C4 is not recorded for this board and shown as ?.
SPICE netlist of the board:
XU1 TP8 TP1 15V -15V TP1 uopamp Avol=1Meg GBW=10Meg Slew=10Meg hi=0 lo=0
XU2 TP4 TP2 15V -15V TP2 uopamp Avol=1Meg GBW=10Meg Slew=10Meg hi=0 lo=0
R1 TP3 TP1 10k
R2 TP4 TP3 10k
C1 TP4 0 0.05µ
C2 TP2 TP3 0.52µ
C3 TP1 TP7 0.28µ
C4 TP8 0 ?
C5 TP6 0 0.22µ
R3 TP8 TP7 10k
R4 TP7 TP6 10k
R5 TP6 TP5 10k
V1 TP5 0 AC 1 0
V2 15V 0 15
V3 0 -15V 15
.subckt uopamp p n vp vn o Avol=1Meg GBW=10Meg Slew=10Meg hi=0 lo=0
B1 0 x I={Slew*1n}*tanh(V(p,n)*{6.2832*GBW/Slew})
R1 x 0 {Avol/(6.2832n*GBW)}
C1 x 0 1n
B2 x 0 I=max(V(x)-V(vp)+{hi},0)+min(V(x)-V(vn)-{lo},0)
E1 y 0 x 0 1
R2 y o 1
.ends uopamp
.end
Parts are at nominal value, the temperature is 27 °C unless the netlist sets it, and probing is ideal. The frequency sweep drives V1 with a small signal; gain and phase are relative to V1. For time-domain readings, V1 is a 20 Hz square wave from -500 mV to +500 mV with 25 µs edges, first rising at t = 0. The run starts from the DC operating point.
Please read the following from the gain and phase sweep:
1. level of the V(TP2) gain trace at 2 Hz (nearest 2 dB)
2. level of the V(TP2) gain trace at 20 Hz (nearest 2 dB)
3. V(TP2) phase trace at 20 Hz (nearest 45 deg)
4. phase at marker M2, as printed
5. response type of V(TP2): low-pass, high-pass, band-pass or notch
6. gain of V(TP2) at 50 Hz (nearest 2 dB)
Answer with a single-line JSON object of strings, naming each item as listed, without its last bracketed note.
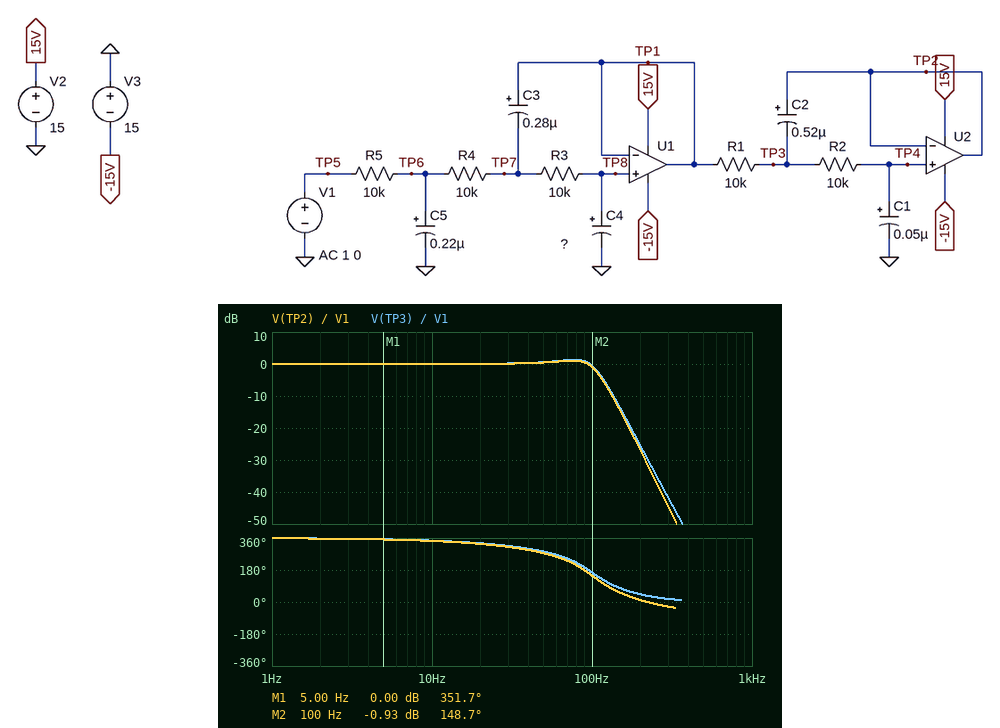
{"level of the V(TP2) gain trace at 2 Hz": "0 dB", "level of the V(TP2) gain trace at 20 Hz": "0 dB", "V(TP2) phase trace at 20 Hz": "315 deg", "phase at marker M2, as printed": "148.7 deg", "response type of V(TP2): low-pass, high-pass, band-pass or notch": "low-pass", "gain of V(TP2) at 50 Hz": "0 dB"}
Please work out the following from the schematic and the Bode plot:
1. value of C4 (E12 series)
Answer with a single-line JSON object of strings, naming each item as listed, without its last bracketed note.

{"value of C4": "47 nF"}
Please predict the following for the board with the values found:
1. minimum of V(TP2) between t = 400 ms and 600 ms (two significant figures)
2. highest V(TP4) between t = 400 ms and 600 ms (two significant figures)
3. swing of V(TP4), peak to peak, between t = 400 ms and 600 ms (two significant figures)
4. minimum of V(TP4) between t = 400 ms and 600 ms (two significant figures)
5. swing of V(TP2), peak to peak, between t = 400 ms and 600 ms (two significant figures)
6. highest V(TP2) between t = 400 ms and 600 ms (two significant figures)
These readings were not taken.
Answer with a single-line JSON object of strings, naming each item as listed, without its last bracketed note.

{"minimum of V(TP2) between t = 400 ms and 600 ms": "-680 mV", "highest V(TP4) between t = 400 ms and 600 ms": "680 mV", "swing of V(TP4), peak to peak, between t = 400 ms and 600 ms": "1.4 V", "minimum of V(TP4) between t = 400 ms and 600 ms": "-680 mV", "swing of V(TP2), peak to peak, between t = 400 ms and 600 ms": "1.4 V", "highest V(TP2) between t = 400 ms and 600 ms": "680 mV"}
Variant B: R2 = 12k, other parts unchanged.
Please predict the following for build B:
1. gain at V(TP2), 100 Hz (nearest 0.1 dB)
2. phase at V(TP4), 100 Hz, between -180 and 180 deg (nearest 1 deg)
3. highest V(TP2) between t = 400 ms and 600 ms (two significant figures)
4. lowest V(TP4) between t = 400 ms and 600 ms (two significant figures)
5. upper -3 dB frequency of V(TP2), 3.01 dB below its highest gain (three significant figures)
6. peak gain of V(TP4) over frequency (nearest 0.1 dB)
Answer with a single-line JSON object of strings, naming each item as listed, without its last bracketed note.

{"gain at V(TP2), 100 Hz": "-2.2 dB", "phase at V(TP4), 100 Hz, between -180 and 180 deg": "133 deg", "highest V(TP2) between t = 400 ms and 600 ms": "700 mV", "lowest V(TP4) between t = 400 ms and 600 ms": "-700 mV", "upper -3 dB frequency of V(TP2), 3.01 dB below its highest gain": "97.2 Hz", "peak gain of V(TP4) over frequency": "1.5 dB"}
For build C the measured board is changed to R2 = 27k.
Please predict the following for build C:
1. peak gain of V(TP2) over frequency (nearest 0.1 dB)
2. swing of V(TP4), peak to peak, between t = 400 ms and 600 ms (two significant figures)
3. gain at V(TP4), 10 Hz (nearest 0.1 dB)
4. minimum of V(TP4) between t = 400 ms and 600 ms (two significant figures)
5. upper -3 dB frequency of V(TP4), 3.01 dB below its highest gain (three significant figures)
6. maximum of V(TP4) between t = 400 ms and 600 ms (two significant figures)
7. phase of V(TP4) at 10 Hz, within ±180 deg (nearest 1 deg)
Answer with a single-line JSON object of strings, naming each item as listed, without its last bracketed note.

{"peak gain of V(TP2) over frequency": "2.3 dB", "swing of V(TP4), peak to peak, between t = 400 ms and 600 ms": "1.5 V", "gain at V(TP4), 10 Hz": "0.1 dB", "minimum of V(TP4) between t = 400 ms and 600 ms": "-740 mV", "upper -3 dB frequency of V(TP4), 3.01 dB below its highest gain": "67.5 Hz", "maximum of V(TP4) between t = 400 ms and 600 ms": "740 mV", "phase of V(TP4) at 10 Hz, within ±180 deg": "-20 deg"}
